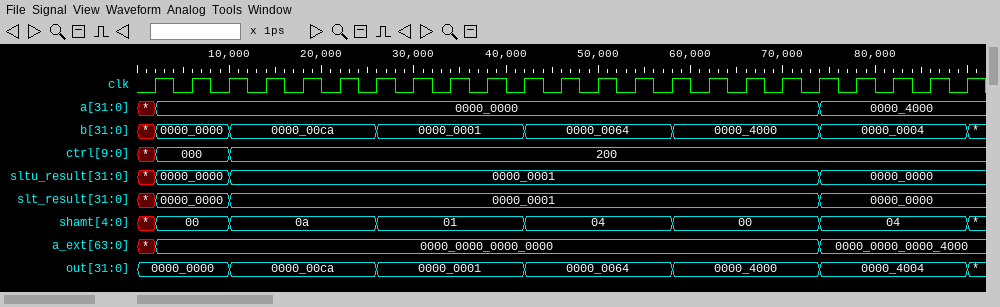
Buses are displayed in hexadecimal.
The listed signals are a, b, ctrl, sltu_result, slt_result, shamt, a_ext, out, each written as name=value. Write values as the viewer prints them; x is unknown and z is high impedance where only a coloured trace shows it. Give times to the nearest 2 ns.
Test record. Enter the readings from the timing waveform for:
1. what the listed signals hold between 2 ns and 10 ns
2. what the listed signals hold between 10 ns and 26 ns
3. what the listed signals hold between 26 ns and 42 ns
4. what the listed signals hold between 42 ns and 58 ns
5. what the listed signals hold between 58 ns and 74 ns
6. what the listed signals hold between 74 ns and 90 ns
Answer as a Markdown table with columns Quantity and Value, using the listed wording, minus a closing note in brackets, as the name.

| Quantity | Value |
|---|---|
| what the listed signals hold between 2 ns and 10 ns | a=0000_0000, b=0000_0000, ctrl=000, sltu_result=0000_0000, slt_result=0000_0000, shamt=00, a_ext=0000_0000_0000_0000, out=0000_0000 |
| what the listed signals hold between 10 ns and 26 ns | a=0000_0000, b=0000_00ca, ctrl=200, sltu_result=0000_0001, slt_result=0000_0001, shamt=0a, a_ext=0000_0000_0000_0000, out=0000_00ca |
| what the listed signals hold between 26 ns and 42 ns | a=0000_0000, b=0000_0001, ctrl=200, sltu_result=0000_0001, slt_result=0000_0001, shamt=01, a_ext=0000_0000_0000_0000, out=0000_0001 |
| what the listed signals hold between 42 ns and 58 ns | a=0000_0000, b=0000_0064, ctrl=200, sltu_result=0000_0001, slt_result=0000_0001, shamt=04, a_ext=0000_0000_0000_0000, out=0000_0064 |
| what the listed signals hold between 58 ns and 74 ns | a=0000_0000, b=0000_4000, ctrl=200, sltu_result=0000_0001, slt_result=0000_0001, shamt=00, a_ext=0000_0000_0000_0000, out=0000_4000 |
| what the listed signals hold between 74 ns and 90 ns | a=0000_4000, b=0000_0004, ctrl=200, sltu_result=0000_0000, slt_result=0000_0000, shamt=04, a_ext=0000_0000_0000_4000, out=0000_4004 |
